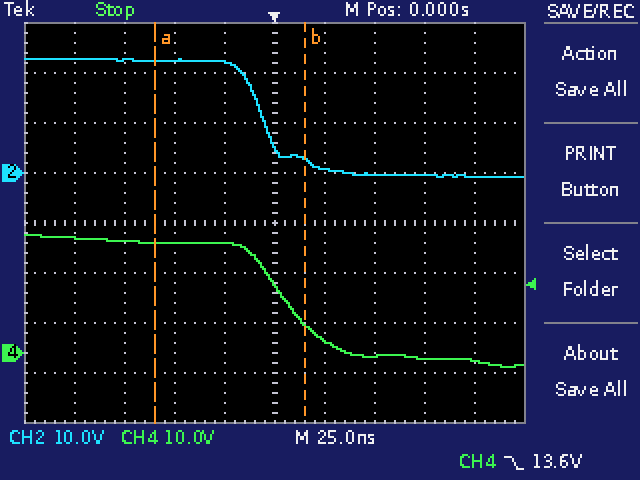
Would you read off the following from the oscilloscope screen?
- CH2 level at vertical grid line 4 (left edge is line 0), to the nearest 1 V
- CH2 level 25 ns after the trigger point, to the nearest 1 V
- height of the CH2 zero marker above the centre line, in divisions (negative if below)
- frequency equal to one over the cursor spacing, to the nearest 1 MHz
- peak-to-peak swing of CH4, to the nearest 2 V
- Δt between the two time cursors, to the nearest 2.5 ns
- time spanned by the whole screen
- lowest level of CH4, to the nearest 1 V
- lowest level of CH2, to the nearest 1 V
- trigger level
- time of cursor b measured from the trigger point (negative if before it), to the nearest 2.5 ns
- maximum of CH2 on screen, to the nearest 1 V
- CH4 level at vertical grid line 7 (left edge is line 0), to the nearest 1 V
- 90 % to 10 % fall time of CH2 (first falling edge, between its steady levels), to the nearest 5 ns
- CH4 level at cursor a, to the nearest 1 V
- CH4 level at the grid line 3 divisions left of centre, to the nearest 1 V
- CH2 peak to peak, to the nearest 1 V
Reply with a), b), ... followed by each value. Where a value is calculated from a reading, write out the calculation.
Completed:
a) 22 V
b) 1 V
c) +1.0 div
d) 1 / 75.0 ns ≈ 13 MHz
e) 26 V
f) 75.0 ns
g) 250 ns
h) -3 V
i) -1 V
j) 13.6 V
k) +15.0 ns
l) 23 V
m) -1 V
n) 35 ns
o) 22 V
p) 22 V
q) 23 V − (-1 V) = 24 V
